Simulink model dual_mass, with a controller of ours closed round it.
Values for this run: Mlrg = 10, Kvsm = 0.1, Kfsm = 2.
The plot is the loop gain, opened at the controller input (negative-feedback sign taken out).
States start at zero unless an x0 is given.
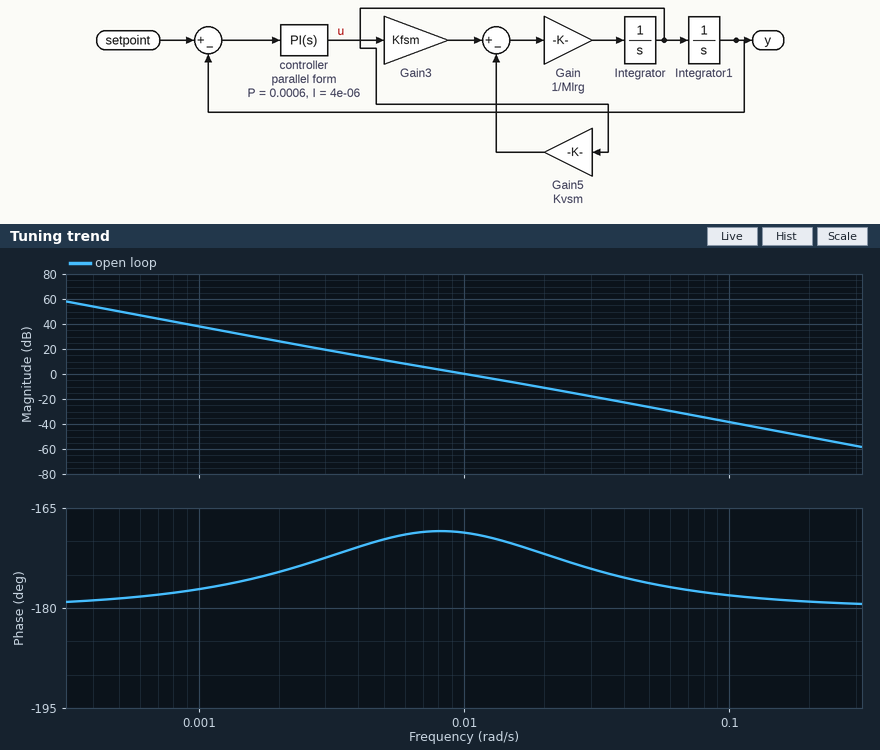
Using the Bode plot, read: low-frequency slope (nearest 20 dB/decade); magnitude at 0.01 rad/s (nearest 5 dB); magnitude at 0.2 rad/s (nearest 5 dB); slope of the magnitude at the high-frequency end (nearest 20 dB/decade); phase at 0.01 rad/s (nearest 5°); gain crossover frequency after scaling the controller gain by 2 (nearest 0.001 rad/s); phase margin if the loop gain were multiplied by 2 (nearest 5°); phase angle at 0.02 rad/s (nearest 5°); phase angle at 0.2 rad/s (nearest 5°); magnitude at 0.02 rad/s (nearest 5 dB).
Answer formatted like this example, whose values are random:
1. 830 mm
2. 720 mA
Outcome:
1. -40 dB/decade
2. 0 dB
3. -50 dB
4. -40 dB/decade
5. -170°
6. 0.015 rad/s
7. 10°
8. -170°
9. -180°
10. -10 dB
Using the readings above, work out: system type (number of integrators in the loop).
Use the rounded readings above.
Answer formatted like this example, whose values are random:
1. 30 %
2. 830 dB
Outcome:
1. 2
